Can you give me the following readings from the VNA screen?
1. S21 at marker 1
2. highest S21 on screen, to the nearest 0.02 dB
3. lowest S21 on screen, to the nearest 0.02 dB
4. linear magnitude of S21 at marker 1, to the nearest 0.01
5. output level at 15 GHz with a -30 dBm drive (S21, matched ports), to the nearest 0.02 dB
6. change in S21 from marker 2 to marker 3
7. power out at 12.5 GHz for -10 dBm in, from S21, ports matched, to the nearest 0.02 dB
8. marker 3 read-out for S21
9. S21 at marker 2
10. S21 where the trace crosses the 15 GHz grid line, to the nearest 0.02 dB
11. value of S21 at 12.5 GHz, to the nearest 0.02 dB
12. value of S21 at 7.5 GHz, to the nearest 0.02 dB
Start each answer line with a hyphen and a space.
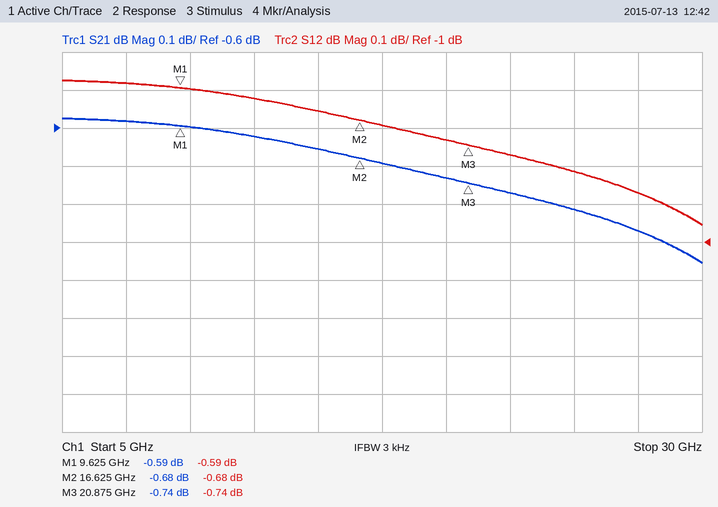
- -0.59 dB
- -0.58 dB
- -0.96 dB
- 0.93
- -30.66 dBm
- -0.06 dB
- -10.62 dBm
- -0.74 dB
- -0.68 dB
- -0.66 dB
- -0.62 dB
- -0.58 dB
